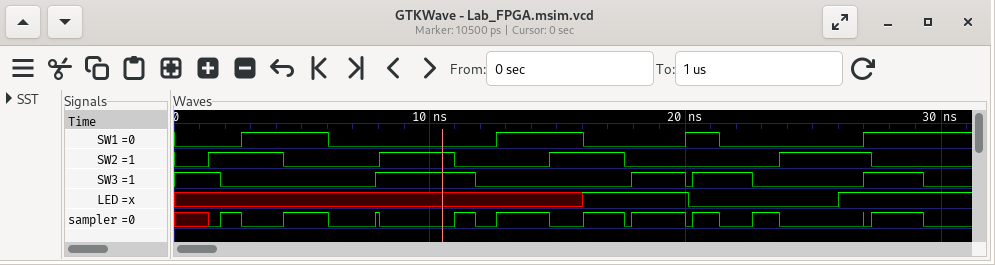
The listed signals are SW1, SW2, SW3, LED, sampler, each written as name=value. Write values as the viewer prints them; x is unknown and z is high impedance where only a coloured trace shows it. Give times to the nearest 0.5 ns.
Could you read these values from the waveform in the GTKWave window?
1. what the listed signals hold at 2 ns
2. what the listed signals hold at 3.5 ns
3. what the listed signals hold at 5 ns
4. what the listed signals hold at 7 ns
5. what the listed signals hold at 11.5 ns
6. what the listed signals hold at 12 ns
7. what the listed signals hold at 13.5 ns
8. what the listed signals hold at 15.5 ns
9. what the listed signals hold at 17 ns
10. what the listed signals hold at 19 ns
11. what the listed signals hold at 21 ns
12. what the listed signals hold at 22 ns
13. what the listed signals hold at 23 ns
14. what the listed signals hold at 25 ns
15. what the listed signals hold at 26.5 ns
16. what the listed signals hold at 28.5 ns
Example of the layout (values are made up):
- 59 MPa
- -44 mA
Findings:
- SW1=0, SW2=1, SW3=0, LED=x, sampler=1
- SW1=1, SW2=1, SW3=0, LED=x, sampler=0
- SW1=1, SW2=0, SW3=0, LED=x, sampler=1
- SW1=0, SW2=0, SW3=0, LED=x, sampler=0
- SW1=0, SW2=0, SW3=1, LED=x, sampler=1
- SW1=0, SW2=0, SW3=0, LED=x, sampler=0
- SW1=1, SW2=0, SW3=0, LED=x, sampler=1
- SW1=1, SW2=1, SW3=0, LED=x, sampler=0
- SW1=0, SW2=1, SW3=0, LED=1, sampler=1
- SW1=0, SW2=0, SW3=1, LED=1, sampler=1
- SW1=1, SW2=0, SW3=1, LED=0, sampler=1
- SW1=0, SW2=0, SW3=1, LED=0, sampler=0
- SW1=0, SW2=0, SW3=0, LED=0, sampler=1
- SW1=0, SW2=1, SW3=0, LED=0, sampler=0
- SW1=0, SW2=1, SW3=0, LED=1, sampler=0
- SW1=1, SW2=0, SW3=1, LED=1, sampler=1
